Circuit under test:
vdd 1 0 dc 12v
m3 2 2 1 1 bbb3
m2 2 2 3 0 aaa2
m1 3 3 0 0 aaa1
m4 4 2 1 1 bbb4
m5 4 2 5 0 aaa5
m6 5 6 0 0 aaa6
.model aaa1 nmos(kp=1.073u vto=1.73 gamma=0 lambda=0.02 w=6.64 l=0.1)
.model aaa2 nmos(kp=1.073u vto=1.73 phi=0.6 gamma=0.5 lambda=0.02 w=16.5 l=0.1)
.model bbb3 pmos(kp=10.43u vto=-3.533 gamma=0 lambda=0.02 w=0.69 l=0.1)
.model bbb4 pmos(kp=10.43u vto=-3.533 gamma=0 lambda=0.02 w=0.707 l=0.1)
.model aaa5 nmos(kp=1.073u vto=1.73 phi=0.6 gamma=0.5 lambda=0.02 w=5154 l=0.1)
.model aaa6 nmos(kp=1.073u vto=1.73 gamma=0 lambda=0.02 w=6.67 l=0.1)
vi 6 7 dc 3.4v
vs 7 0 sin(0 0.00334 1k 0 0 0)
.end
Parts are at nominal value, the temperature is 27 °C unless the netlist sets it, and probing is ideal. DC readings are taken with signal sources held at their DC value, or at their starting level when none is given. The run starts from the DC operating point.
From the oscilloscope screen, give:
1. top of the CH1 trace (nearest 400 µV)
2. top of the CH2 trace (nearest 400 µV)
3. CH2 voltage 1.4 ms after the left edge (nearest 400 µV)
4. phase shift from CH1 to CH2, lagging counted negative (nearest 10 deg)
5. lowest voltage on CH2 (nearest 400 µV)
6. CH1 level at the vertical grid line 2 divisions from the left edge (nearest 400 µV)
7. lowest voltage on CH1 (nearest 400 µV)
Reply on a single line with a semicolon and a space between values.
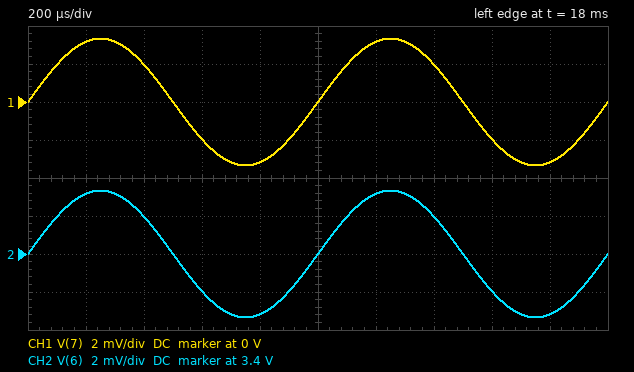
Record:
3.2 mV; 3.4032 V; 3.4020 V; 0 deg; 3.3968 V; 2.0 mV; -3.2 mV
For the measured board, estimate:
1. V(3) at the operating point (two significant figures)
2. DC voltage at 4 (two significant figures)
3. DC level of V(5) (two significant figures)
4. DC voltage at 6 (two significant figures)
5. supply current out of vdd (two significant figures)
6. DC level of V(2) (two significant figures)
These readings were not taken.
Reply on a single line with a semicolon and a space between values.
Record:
3.4 V; 7.7 V; 4.3 V; 3.4 V; 220 µA; 6.8 V
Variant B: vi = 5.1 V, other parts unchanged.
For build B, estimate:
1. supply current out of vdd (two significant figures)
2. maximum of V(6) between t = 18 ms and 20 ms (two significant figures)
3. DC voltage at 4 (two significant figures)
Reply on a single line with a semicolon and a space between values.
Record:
230 µA; 5.1 V; 550 mV
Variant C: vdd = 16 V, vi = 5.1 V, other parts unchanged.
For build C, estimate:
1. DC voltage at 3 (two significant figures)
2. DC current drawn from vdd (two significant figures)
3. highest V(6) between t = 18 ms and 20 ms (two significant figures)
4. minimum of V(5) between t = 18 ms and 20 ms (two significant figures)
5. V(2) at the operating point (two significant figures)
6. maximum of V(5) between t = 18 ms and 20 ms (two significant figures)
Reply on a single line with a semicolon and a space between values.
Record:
4.9 V; 820 µA; 5.1 V; 3.6 V; 9.4 V; 3.7 V
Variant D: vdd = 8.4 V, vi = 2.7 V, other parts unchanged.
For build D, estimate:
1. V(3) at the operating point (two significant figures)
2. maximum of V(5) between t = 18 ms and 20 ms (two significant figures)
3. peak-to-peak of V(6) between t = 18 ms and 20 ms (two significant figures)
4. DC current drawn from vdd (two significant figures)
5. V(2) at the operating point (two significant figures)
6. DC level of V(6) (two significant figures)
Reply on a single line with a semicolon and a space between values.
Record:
2.1 V; 86 mV; 6.7 mV; 11 µA; 4.5 V; 2.7 V
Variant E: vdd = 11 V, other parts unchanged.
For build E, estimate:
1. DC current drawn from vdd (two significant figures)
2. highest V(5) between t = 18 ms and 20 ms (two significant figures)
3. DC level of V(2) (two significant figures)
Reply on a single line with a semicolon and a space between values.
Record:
140 µA; 800 mV; 6.2 V
